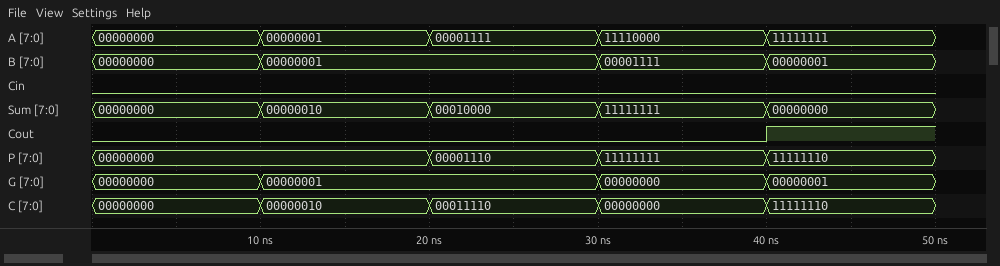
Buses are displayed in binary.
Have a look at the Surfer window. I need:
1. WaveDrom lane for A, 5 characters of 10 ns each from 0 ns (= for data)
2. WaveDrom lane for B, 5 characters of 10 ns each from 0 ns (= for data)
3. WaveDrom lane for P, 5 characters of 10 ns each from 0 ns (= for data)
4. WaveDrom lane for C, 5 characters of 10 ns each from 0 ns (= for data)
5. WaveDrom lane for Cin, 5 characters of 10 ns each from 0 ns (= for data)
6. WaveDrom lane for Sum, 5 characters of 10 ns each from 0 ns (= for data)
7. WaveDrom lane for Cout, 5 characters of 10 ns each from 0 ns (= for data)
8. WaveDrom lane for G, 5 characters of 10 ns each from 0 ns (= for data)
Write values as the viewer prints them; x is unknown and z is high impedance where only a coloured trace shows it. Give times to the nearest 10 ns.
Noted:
{name: 'A', wave: '=====', data: '00000000 00000001 00001111 11110000 11111111'}
{name: 'B', wave: '==.==', data: '00000000 00000001 00001111 00000001'}
{name: 'P', wave: '=.===', data: '00000000 00001110 11111111 11111110'}
{name: 'C', wave: '=====', data: '00000000 00000010 00011110 00000000 11111110'}
{name: 'Cin', wave: '0....'}
{name: 'Sum', wave: '=====', data: '00000000 00000010 00010000 11111111 00000000'}
{name: 'Cout', wave: '0...1'}
{name: 'G', wave: '==.==', data: '00000000 00000001 00000000 00000001'}
